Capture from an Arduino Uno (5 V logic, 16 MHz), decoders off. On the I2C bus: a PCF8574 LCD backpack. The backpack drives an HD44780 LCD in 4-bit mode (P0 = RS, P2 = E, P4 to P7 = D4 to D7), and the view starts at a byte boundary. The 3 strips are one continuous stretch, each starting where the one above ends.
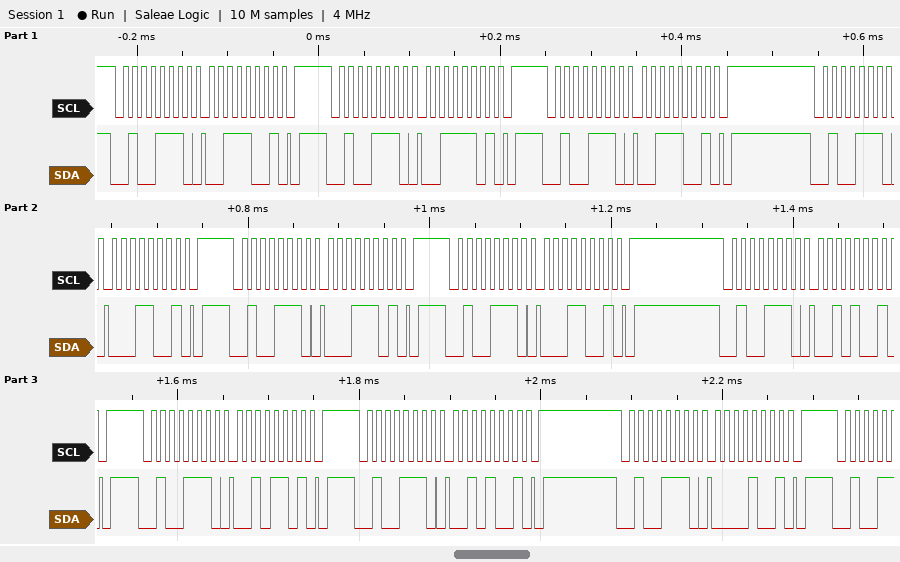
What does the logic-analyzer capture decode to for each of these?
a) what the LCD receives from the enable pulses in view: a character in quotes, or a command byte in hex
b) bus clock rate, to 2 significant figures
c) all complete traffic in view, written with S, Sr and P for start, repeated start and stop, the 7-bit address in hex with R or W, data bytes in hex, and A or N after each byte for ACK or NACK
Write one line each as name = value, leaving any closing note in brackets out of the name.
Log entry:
what the LCD receives from the enable pulses in view: a character in quotes, or a command byte in hex = '1'
bus clock rate, to 2 significant figures = 100 kHz
all complete traffic in view, written with S, Sr and P for start, repeated start and stop, the 7-bit address in hex with R or W, data bytes in hex, and A or N after each byte for ACK or NACK = S 27W A 39 A P S 27W A 3D A P S 27W A 39 A P S 27W A 19 A P S 27W A 1D A P S 27W A 19 A P S 27W A 29 A P S 27W A 2D A P S 27W A 29 A P S 27W A 09 A P
